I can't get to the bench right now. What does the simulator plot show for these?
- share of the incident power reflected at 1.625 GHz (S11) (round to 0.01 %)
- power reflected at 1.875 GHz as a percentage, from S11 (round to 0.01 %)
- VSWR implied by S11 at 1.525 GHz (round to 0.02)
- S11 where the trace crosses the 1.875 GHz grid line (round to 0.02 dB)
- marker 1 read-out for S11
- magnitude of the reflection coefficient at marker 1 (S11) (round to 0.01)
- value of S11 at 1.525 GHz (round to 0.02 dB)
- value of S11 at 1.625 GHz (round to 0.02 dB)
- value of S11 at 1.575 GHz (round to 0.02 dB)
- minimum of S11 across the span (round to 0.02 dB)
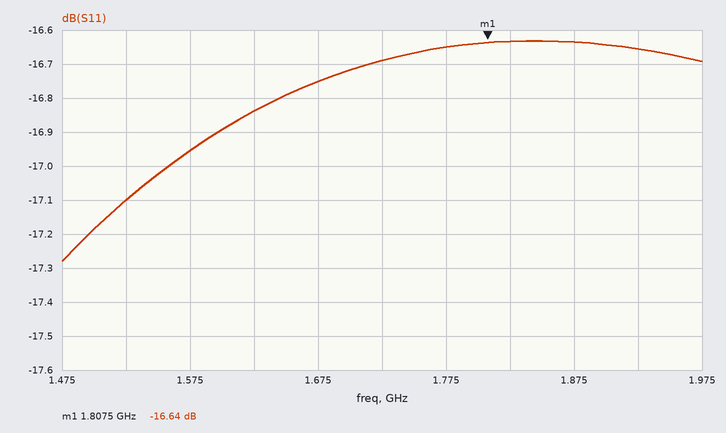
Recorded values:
2.07 %
2.17 %
1.32
-16.64 dB
-16.64 dB
0.15
-17.10 dB
-16.84 dB
-16.96 dB
-17.28 dB
